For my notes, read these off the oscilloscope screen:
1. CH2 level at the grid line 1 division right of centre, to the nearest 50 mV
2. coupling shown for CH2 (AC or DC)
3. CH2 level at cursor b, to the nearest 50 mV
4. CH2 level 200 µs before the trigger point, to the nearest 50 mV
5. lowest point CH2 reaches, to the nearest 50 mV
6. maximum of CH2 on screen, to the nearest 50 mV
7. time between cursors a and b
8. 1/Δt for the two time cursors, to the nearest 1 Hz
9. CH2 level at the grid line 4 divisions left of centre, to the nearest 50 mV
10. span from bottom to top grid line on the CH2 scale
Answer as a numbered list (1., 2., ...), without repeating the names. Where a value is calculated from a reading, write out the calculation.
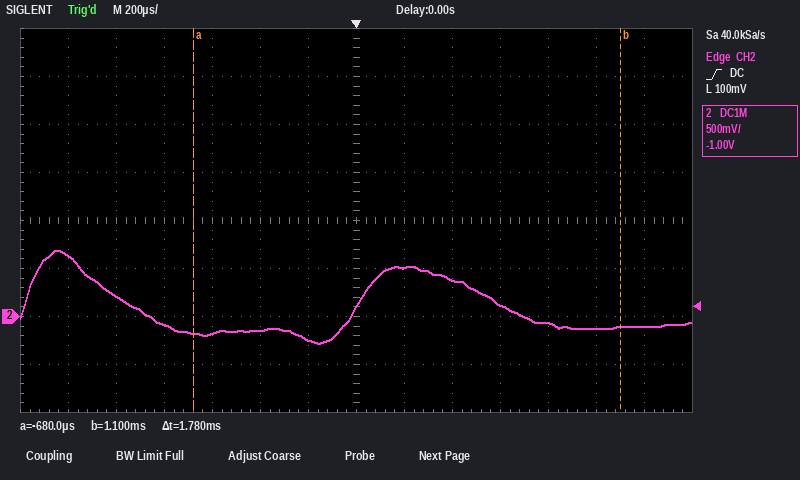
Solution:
1. 500 mV
2. DC
3. -100 mV
4. -250 mV
5. -300 mV
6. 700 mV
7. 1.78 ms
8. 1 / 1.78 ms ≈ 562 Hz
9. -100 mV
10. 4 V
